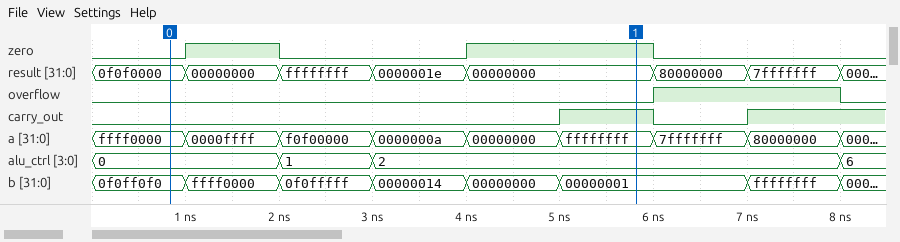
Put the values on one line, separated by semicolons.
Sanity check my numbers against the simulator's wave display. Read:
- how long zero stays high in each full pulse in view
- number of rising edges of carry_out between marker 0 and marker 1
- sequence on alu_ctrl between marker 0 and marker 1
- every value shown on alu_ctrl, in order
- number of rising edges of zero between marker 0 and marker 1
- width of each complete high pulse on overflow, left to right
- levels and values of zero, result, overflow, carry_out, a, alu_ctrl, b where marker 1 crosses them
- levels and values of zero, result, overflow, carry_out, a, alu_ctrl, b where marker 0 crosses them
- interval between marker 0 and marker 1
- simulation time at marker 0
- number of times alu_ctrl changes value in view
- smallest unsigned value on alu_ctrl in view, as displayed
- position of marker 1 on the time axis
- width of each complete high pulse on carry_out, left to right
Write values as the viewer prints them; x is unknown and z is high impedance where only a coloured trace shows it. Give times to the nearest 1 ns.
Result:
1 ns, 2 ns; 1; 0, 1, 2; 0, 1, 2, 6; 2; 2 ns; zero=1, result=00000000, overflow=0, carry_out=1, a=ffffffff, alu_ctrl=2, b=00000001; zero=0, result=0f0f0000, overflow=0, carry_out=0, a=ffff0000, alu_ctrl=0, b=0f0ff0f0; 5 ns; 1 ns; 3; 0; 6 ns; 1 ns
